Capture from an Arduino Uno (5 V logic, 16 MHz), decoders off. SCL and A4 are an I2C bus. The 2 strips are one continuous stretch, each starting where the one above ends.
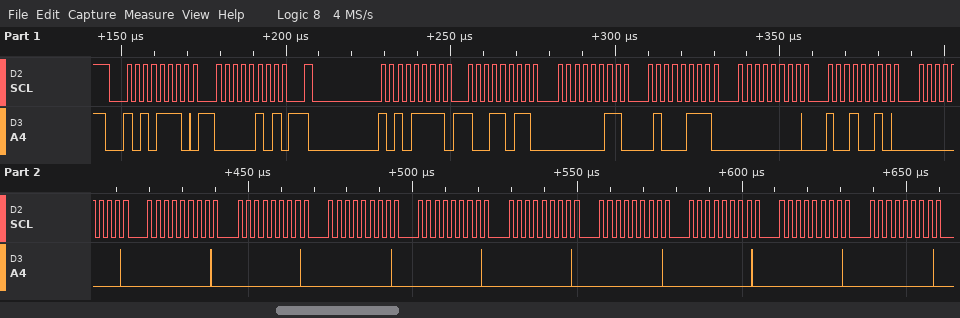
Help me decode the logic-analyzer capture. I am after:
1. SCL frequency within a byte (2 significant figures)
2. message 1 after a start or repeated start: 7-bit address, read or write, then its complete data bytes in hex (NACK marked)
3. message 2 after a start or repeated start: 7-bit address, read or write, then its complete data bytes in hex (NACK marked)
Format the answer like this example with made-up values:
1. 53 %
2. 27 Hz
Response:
1. 400 kHz
2. 0x57 write: 05
3. 0x57 read: 9B 03 47 00 92 00 00 00 00 00 00 00 00 00 00
